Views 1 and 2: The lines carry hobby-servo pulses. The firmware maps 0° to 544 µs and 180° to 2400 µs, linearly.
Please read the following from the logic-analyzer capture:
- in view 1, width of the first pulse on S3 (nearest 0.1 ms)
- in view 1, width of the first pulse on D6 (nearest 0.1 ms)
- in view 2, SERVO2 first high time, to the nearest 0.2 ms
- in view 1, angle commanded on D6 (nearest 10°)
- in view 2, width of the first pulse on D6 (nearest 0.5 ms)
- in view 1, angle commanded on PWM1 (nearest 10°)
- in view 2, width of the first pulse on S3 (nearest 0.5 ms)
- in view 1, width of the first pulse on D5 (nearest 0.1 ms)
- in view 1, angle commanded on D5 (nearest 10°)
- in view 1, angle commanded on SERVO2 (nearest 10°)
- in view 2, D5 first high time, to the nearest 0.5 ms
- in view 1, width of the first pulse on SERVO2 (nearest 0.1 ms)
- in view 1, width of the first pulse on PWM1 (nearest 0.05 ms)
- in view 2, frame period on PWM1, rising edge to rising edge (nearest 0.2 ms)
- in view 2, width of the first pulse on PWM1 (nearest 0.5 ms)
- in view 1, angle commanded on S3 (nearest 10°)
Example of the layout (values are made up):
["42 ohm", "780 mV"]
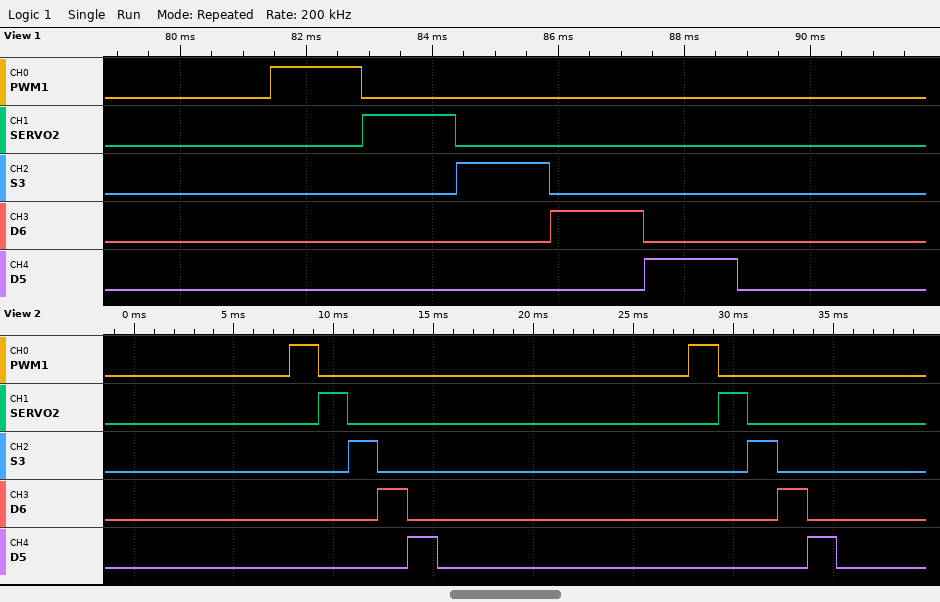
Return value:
["1.5 ms", "1.5 ms", "1.4 ms", "90°", "1.5 ms", "90°", "1.5 ms", "1.5 ms", "90°", "90°", "1.5 ms", "1.5 ms", "1.45 ms", "20.0 ms", "1.5 ms", "90°"]
